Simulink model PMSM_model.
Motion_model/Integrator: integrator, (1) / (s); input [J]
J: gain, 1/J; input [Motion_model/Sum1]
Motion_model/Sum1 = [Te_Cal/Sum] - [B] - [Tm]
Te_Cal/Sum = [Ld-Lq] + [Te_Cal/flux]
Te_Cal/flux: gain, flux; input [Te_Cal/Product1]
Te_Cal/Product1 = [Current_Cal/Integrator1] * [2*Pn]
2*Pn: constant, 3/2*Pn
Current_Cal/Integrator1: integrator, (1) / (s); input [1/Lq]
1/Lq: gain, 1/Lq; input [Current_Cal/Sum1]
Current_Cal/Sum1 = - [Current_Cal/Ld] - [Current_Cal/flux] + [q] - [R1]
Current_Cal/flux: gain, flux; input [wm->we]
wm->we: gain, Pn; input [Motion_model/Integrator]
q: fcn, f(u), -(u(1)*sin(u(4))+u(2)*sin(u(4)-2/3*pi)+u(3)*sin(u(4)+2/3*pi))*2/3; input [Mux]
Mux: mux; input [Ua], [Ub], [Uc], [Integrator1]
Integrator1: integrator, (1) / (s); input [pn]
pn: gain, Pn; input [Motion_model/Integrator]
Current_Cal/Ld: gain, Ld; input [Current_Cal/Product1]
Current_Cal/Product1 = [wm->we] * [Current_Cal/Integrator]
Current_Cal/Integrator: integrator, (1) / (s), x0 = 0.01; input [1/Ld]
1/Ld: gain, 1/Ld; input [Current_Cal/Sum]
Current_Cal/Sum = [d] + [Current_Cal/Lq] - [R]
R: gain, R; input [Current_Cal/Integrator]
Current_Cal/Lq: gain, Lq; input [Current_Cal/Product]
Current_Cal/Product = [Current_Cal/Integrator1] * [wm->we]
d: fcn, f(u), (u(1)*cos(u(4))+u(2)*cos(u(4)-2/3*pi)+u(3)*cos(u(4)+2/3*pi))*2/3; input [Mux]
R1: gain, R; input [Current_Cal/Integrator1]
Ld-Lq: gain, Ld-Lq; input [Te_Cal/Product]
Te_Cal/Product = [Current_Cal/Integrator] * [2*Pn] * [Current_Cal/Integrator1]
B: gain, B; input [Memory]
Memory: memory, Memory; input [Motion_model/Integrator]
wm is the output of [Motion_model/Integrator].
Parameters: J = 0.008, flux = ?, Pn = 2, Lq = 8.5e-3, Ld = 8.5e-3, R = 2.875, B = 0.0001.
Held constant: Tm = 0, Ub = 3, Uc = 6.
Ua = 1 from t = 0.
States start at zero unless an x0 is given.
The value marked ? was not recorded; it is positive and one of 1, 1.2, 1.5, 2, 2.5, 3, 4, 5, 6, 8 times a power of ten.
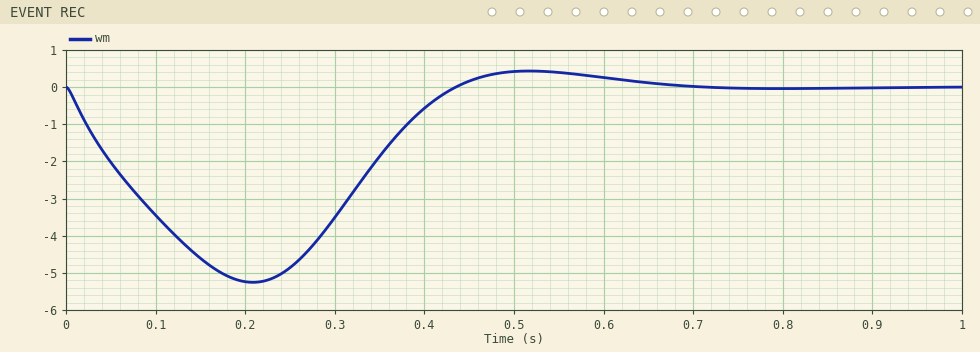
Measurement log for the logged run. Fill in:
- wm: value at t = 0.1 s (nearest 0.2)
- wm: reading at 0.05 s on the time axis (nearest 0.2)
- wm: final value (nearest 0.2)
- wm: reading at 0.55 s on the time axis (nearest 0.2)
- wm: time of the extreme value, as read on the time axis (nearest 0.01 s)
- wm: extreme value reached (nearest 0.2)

-3.4
-2.0
0.0
0.4
0.21 s
-5.2
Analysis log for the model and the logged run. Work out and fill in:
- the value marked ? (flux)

0.25
